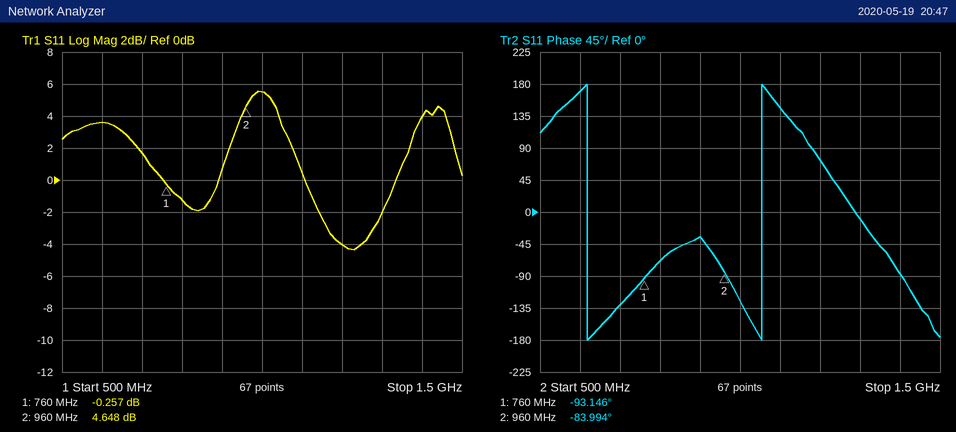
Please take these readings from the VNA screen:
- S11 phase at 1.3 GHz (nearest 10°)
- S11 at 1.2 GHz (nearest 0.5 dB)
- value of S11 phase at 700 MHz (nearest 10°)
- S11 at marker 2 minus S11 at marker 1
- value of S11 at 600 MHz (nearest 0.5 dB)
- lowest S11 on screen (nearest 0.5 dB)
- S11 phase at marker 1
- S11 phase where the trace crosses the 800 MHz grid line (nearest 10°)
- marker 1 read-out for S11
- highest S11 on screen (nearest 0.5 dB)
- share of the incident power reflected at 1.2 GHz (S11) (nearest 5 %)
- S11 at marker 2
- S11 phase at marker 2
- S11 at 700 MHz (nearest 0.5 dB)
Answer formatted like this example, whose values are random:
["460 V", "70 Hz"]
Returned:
["-10°", "-4.0 dB", "-130°", "4.905 dB", "3.5 dB", "-4.5 dB", "-93.146°", "-70°", "-0.257 dB", "5.5 dB", "40 %", "4.648 dB", "-83.994°", "1.5 dB"]
